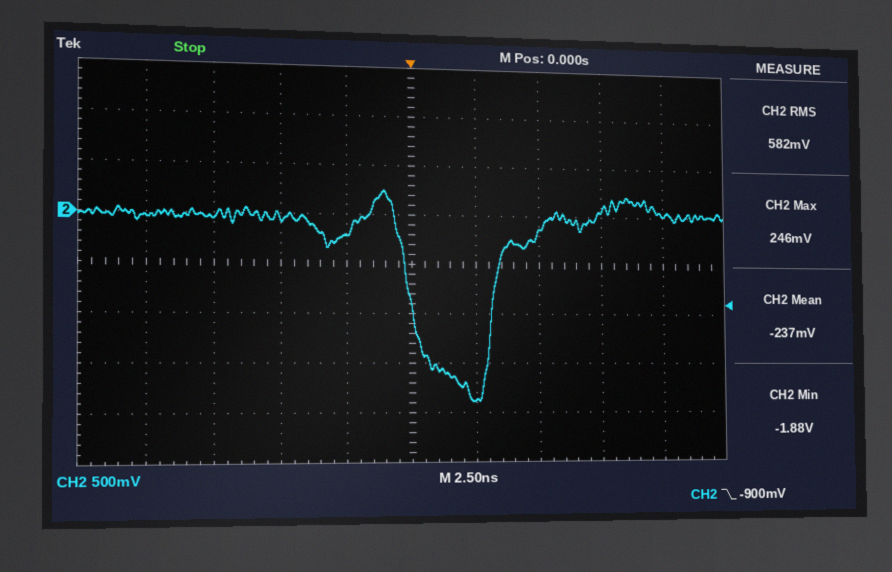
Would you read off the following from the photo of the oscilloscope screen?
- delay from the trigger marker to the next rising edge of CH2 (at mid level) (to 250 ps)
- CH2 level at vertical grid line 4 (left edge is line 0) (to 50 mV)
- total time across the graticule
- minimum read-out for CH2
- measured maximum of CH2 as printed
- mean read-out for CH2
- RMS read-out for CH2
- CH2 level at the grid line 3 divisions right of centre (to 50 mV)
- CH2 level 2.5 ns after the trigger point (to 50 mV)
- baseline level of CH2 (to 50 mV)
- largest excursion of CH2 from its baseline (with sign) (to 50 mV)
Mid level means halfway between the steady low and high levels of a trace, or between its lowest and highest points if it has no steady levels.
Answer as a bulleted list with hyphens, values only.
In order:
- 3.25 ns
- -200 mV
- 25 ns
- -1.88 V
- 246 mV
- -237 mV
- 582 mV
- 100 mV
- -1.85 V
- 0 mV
- -1.85 V
